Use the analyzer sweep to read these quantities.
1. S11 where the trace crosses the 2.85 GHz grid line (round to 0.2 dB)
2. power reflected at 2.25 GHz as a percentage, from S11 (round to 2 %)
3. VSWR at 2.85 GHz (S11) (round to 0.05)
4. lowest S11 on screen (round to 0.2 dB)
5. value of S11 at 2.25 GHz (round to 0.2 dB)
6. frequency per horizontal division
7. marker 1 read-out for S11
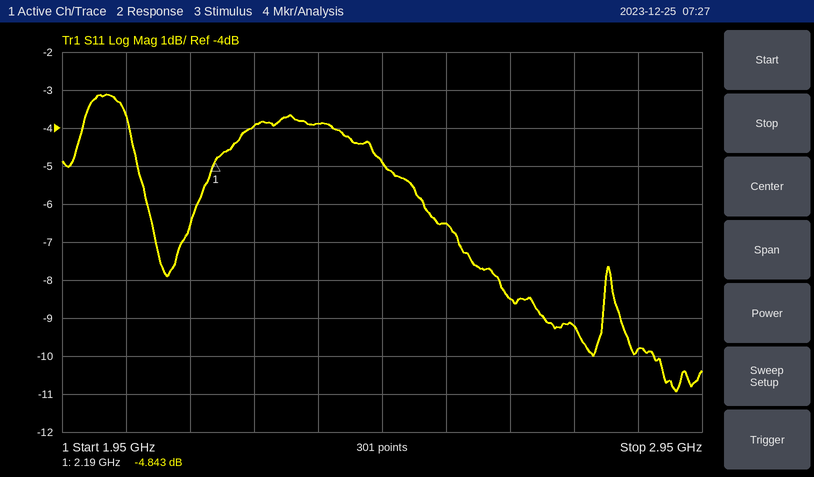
-9.8 dB
40 %
1.95
-11.0 dB
-4.0 dB
100 MHz
-4.843 dB
